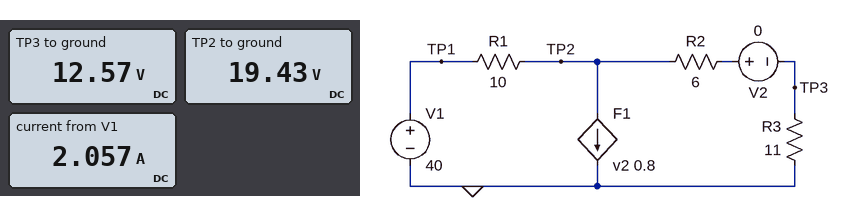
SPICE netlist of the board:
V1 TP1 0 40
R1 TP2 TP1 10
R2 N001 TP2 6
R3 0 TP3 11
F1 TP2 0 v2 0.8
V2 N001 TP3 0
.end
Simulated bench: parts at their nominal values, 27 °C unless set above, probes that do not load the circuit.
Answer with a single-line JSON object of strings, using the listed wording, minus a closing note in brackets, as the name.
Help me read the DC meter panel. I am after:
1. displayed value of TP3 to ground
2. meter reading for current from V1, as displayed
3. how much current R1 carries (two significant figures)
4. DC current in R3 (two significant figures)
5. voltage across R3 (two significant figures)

{"displayed value of TP3 to ground": "12.57 V", "meter reading for current from V1, as displayed": "2.057 A", "how much current R1 carries": "2.1 A", "DC current in R3": "1.1 A", "voltage across R3": "13 V"}
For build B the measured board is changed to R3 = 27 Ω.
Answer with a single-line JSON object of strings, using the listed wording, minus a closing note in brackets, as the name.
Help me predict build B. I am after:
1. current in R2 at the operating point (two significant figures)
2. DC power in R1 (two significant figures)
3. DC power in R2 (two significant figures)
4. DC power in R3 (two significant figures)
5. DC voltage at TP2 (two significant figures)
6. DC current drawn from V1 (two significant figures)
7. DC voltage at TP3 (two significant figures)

{"current in R2 at the operating point": "780 mA", "DC power in R1": "20 W", "DC power in R2": "3.7 W", "DC power in R3": "17 W", "DC voltage at TP2": "26 V", "DC current drawn from V1": "1.4 A", "DC voltage at TP3": "21 V"}
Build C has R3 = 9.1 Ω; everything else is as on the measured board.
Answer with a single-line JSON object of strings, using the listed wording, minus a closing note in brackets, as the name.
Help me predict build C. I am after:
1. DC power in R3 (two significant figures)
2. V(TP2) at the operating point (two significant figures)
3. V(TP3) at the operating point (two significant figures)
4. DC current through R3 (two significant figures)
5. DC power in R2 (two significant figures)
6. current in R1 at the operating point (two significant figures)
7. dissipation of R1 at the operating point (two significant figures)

{"DC power in R3": "13 W", "V(TP2) at the operating point": "18 V", "V(TP3) at the operating point": "11 V", "DC current through R3": "1.2 A", "DC power in R2": "8.8 W", "current in R1 at the operating point": "2.2 A", "dissipation of R1 at the operating point": "47 W"}
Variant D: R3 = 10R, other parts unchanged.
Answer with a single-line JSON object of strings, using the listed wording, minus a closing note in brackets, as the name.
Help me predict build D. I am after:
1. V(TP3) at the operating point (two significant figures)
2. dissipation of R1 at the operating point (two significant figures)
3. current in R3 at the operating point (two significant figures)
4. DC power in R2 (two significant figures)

{"V(TP3) at the operating point": "12 V", "dissipation of R1 at the operating point": "45 W", "current in R3 at the operating point": "1.2 A", "DC power in R2": "8.3 W"}
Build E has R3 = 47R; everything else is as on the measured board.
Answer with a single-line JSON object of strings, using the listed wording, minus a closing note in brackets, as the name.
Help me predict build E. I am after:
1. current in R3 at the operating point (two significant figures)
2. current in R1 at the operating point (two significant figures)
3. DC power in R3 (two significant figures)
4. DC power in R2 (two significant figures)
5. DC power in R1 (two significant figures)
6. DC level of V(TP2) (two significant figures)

{"current in R3 at the operating point": "560 mA", "current in R1 at the operating point": "1.0 A", "DC power in R3": "15 W", "DC power in R2": "1.9 W", "DC power in R1": "10 W", "DC level of V(TP2)": "30 V"}
